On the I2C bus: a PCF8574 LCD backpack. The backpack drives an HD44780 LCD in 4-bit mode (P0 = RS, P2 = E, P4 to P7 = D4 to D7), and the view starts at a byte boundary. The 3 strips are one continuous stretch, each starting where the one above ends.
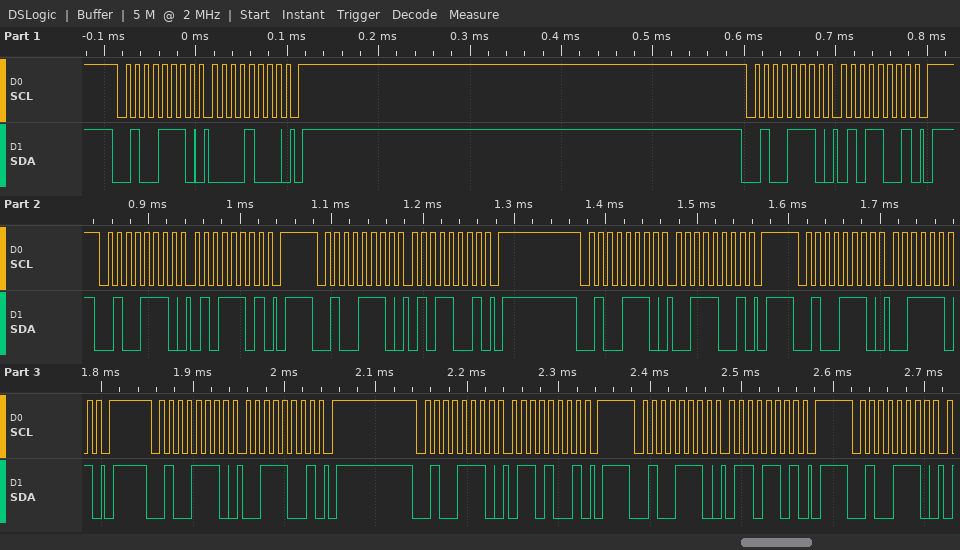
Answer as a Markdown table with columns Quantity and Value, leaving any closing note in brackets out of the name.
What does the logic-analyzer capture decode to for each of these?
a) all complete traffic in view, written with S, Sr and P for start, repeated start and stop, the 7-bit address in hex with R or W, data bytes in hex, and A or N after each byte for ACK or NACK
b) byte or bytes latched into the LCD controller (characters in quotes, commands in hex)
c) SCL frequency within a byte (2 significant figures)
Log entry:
| Quantity | Value |
|---|---|
| all complete traffic in view, written with S, Sr and P for start, repeated start and stop, the 7-bit address in hex with R or W, data bytes in hex, and A or N after each byte for ACK or NACK | S 27W A 08 A P S 27W A 59 A P S 27W A 5D A P S 27W A 59 A P S 27W A 39 A P S 27W A 3D A P S 27W A 39 A P S 27W A 69 A P S 27W A 6D A P S 27W A |
| byte or bytes latched into the LCD controller | 'S' |
| SCL frequency within a byte | 100 kHz |
